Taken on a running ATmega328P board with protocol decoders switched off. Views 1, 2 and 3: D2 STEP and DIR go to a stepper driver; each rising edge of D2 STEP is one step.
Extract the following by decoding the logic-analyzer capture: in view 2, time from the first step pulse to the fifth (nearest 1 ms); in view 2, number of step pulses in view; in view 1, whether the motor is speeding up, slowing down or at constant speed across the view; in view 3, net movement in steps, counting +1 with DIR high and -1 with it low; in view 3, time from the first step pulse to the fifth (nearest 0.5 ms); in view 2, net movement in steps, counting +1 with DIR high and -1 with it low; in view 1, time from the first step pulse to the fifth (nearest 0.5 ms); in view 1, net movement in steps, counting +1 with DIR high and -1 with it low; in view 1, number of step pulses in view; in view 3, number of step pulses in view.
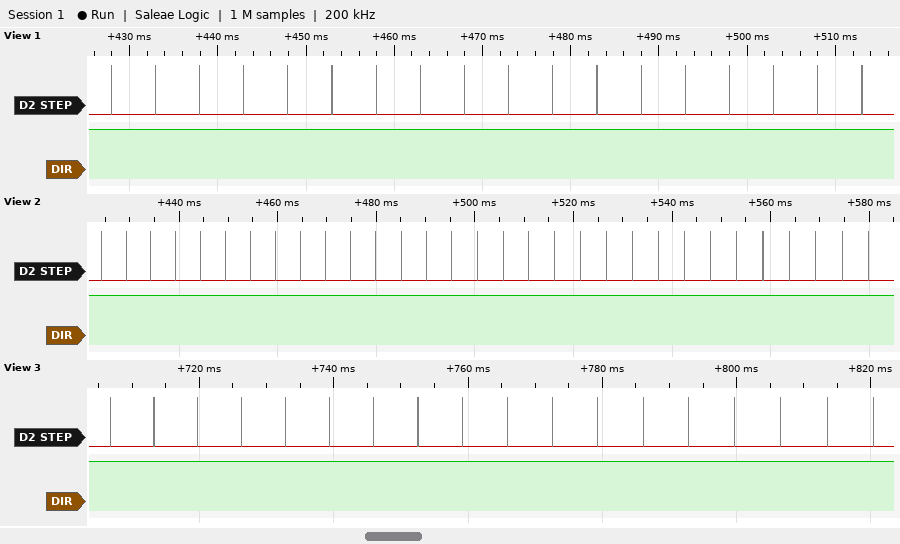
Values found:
20 ms
31
constant speed
+18
26.0 ms
+31
20.0 ms
+18
18
18
